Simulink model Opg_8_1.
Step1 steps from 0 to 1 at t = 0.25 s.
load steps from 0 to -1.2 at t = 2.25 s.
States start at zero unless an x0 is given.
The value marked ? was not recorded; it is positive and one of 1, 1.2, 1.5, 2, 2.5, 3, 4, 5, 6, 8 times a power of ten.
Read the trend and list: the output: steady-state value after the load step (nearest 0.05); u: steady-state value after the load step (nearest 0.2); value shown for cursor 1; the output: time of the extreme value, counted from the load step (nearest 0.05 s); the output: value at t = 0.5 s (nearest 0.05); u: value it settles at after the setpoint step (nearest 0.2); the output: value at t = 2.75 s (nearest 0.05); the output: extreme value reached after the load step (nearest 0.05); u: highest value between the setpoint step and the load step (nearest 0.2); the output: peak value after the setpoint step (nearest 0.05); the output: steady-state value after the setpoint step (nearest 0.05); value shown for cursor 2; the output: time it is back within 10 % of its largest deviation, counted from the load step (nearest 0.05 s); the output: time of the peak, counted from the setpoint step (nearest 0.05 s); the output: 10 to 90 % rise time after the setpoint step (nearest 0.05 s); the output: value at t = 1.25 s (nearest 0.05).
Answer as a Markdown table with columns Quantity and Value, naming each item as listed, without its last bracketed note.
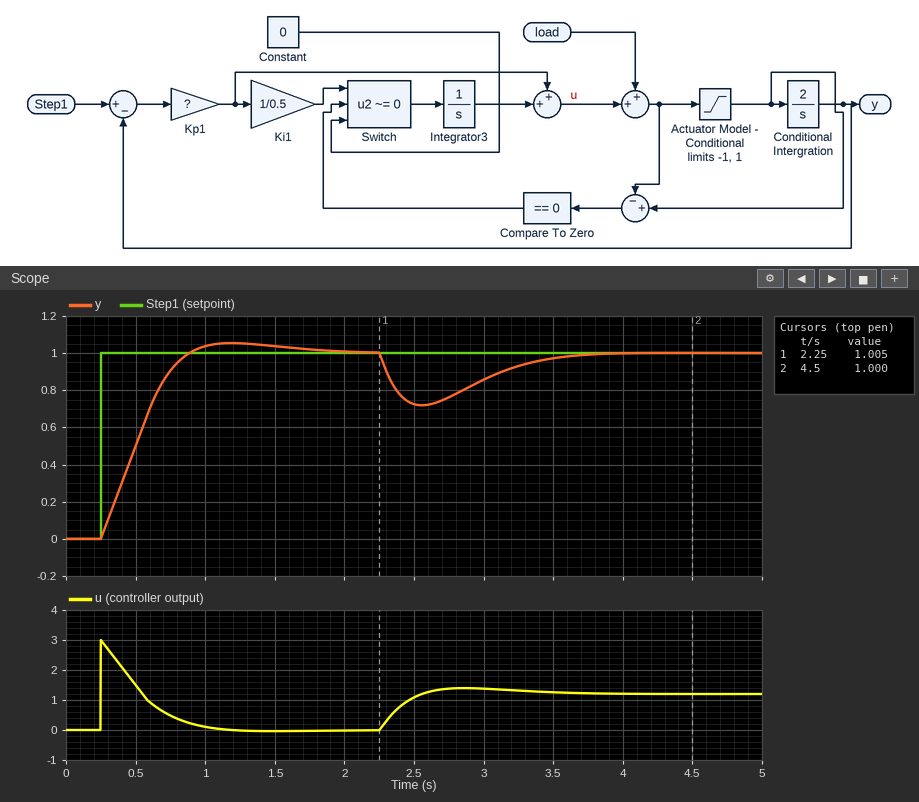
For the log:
| Quantity | Value |
|---|---|
| the output: steady-state value after the load step | 1.00 |
| u: steady-state value after the load step | 1.2 |
| value shown for cursor 1 | 1.005 |
| the output: time of the extreme value, counted from the load step | 0.30 s |
| the output: value at t = 0.5 s | 0.50 |
| u: value it settles at after the setpoint step | 0.0 |
| the output: value at t = 2.75 s | 0.75 |
| the output: extreme value reached after the load step | 0.70 |
| u: highest value between the setpoint step and the load step | 3.0 |
| the output: peak value after the setpoint step | 1.05 |
| the output: steady-state value after the setpoint step | 1.00 |
| value shown for cursor 2 | 1.000 |
| the output: time it is back within 10 % of its largest deviation, counted from the load step | 1.25 s |
| the output: time of the peak, counted from the setpoint step | 0.95 s |
| the output: 10 to 90 % rise time after the setpoint step | 0.45 s |
| the output: value at t = 1.25 s | 1.05 |
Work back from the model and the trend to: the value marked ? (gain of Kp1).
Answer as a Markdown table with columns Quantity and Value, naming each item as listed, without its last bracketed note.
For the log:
| Quantity | Value |
|---|---|
| the value marked ? | 3 |
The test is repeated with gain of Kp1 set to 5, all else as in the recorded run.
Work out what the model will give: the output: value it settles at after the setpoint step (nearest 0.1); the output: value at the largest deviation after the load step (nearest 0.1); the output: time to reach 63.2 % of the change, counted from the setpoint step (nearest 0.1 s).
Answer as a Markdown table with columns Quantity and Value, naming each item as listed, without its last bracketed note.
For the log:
| Quantity | Value |
|---|---|
| the output: value it settles at after the setpoint step | 1.0 |
| the output: value at the largest deviation after the load step | 0.8 |
| the output: time to reach 63.2 % of the change, counted from the setpoint step | 0.3 s |
